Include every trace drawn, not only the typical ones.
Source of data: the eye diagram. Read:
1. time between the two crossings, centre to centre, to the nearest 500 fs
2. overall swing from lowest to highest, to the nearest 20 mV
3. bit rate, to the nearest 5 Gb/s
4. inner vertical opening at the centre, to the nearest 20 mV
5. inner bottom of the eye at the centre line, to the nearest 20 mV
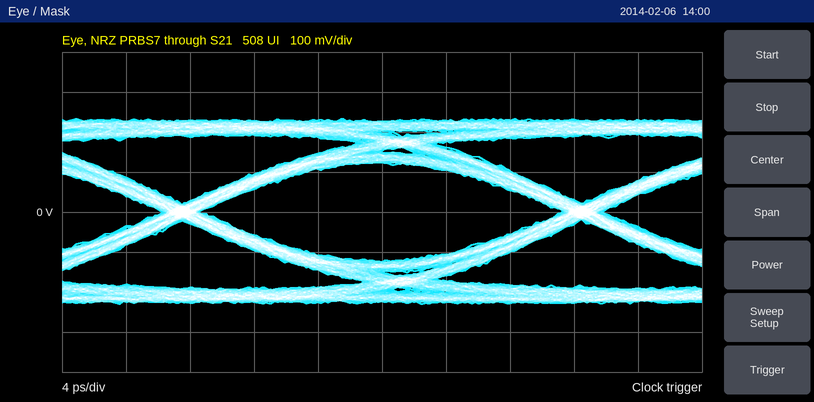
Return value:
25.0 ps
460 mV
40 Gb/s
240 mV
-120 mV
